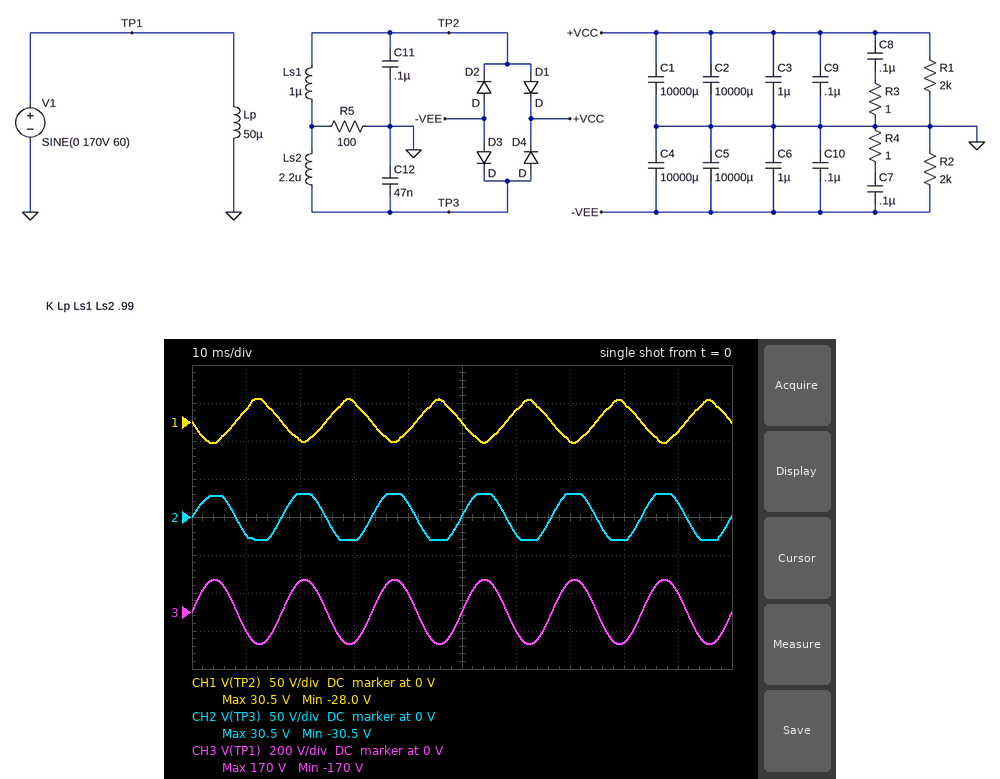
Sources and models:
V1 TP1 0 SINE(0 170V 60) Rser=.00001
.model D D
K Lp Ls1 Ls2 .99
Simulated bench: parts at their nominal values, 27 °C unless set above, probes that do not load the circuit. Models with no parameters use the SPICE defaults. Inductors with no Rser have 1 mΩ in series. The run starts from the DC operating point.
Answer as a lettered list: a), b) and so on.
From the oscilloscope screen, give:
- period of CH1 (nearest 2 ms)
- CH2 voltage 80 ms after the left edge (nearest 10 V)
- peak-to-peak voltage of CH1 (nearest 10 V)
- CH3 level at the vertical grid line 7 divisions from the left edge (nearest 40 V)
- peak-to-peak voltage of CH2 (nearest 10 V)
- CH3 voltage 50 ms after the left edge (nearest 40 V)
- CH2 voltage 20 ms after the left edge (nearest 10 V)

a) 16 ms
b) -30 V
c) 60 V
d) 160 V
e) 60 V
f) 0 V
g) 30 V
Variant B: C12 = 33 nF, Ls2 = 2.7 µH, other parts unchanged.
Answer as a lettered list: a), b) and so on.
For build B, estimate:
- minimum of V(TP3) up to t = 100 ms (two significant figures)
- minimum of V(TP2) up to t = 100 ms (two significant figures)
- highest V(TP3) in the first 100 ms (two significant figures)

a) -33 V
b) -30 V
c) 33 V
